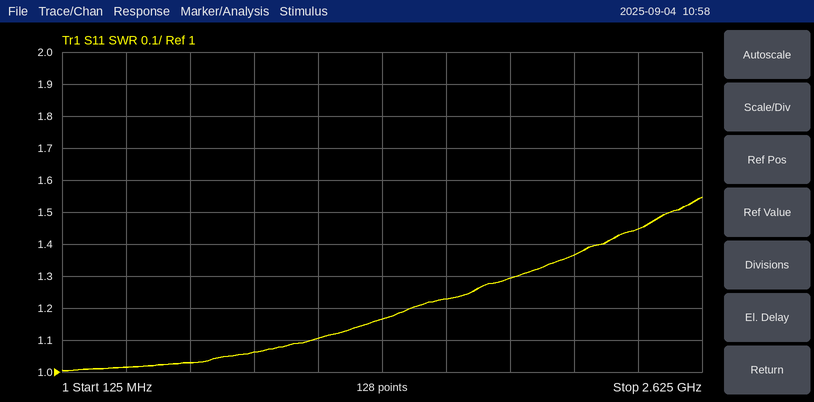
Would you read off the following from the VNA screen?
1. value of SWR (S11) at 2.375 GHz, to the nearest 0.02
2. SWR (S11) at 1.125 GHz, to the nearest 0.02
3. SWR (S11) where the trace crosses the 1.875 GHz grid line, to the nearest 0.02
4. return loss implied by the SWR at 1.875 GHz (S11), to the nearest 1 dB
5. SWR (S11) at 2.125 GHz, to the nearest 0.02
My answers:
1.44
1.10
1.30
18 dB
1.36
